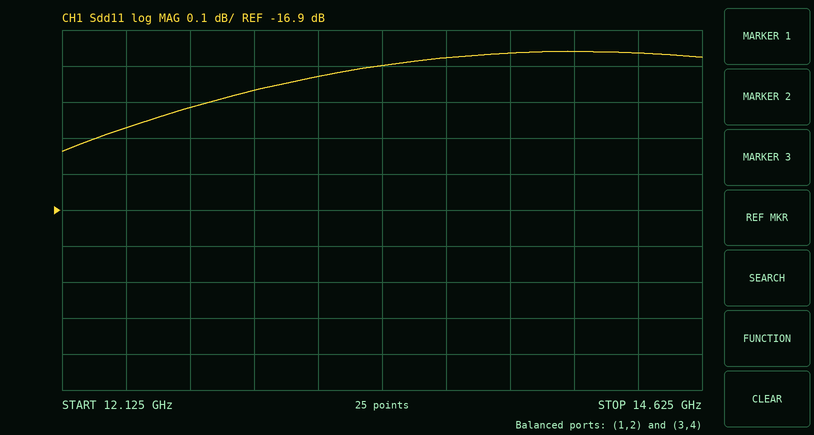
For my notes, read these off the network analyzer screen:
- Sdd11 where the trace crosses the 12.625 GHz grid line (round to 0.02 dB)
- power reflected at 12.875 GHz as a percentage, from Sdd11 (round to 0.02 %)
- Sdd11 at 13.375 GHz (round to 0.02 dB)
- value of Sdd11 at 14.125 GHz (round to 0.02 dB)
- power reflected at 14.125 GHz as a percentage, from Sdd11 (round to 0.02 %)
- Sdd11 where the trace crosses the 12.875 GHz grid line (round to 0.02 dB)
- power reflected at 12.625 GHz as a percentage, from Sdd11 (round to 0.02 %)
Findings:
-16.62 dB
2.20 %
-16.50 dB
-16.46 dB
2.26 %
-16.56 dB
2.18 %
